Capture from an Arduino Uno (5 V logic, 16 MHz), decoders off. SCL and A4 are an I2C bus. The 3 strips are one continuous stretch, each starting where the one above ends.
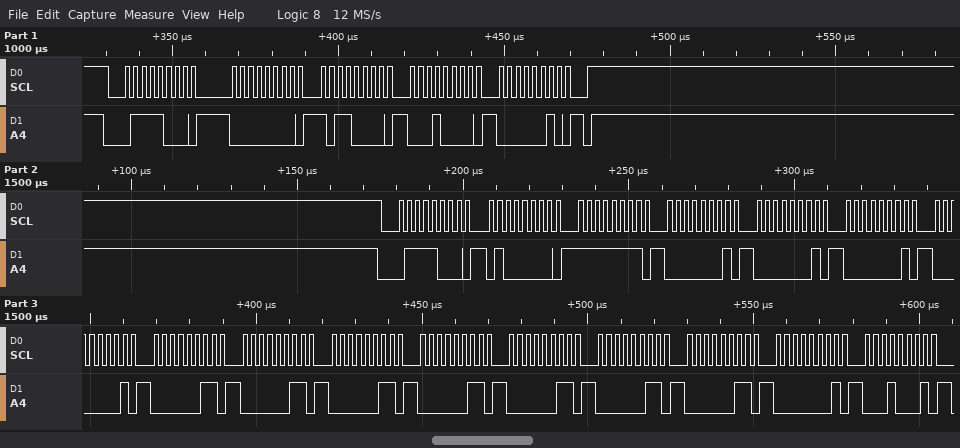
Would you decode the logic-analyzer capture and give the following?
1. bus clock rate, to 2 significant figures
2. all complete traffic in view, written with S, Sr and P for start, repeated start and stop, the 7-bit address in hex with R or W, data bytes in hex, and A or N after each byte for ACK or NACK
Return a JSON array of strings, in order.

["400 kHz", "S 3CW A 00 A B0 A 10 A 02 A P S 3CW A 40 A FF A 01 A 01 A 01 A 01 A 03 A 03 A 03 A 03 A 03 A 03 A 03 A 01 A 11 A"]
